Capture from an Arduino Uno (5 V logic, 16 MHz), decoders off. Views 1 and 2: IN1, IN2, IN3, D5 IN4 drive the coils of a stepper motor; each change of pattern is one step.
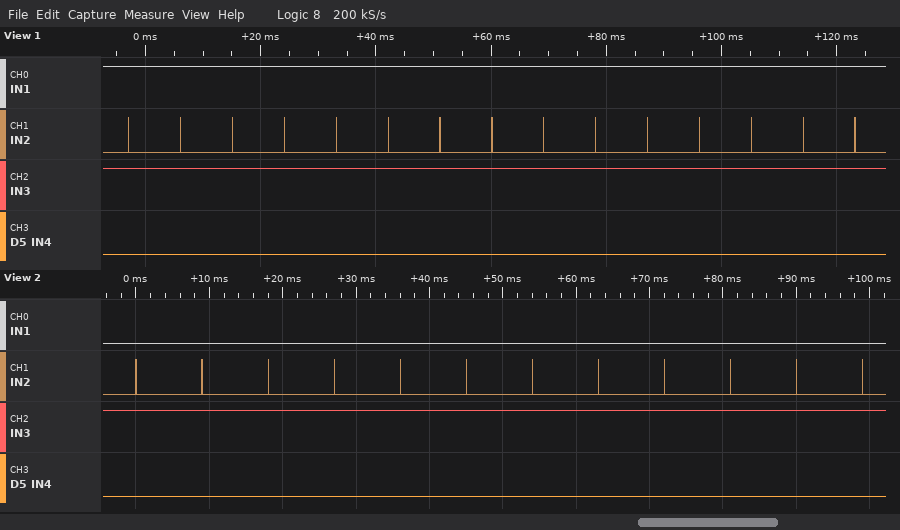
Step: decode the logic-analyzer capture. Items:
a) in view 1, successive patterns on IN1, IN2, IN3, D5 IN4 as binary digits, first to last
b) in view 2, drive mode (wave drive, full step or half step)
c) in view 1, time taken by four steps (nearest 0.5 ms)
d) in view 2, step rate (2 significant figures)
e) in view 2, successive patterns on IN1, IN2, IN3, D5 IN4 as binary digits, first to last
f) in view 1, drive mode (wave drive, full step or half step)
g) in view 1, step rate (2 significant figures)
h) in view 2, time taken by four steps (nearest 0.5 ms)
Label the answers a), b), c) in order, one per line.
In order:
a) 1010 1010 1010 1010 1010 1010 1010 1010 1010 1010 1010 1010 1010 1010 1010 1010
b) wave drive
c) 36.0 ms
d) 110 steps/s
e) 0010 0010 0010 0010 0010 0010 0010 0010 0010 0010 0010 0010 0010
f) full step
g) 110 steps/s
h) 36.0 ms
